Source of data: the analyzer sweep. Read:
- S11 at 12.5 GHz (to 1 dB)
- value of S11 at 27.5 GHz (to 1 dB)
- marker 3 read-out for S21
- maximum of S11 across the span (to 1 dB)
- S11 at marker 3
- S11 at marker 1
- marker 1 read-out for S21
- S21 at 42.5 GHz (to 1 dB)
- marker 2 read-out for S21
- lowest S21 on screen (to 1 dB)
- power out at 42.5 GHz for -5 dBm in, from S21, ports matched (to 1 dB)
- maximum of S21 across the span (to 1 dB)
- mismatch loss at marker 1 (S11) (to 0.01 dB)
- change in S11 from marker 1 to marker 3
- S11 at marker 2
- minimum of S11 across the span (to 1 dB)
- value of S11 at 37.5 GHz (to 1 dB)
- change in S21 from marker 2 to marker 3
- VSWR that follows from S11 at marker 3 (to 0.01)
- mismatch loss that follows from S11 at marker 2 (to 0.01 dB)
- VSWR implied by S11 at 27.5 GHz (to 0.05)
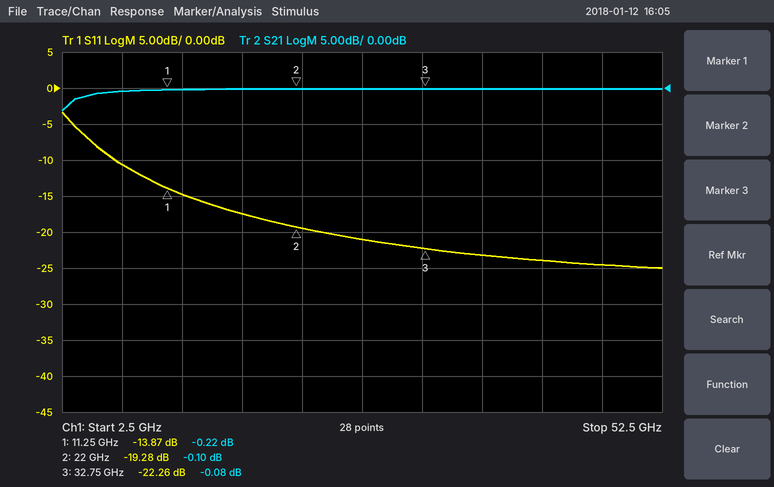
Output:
-15 dB
-21 dB
-0.08 dB
-3 dB
-22.26 dB
-13.87 dB
-0.22 dB
0 dB
-0.10 dB
-3 dB
-5 dBm
0 dB
0.18 dB
-8.39 dB
-19.28 dB
-25 dB
-23 dB
0.02 dB
1.17
0.05 dB
1.20
